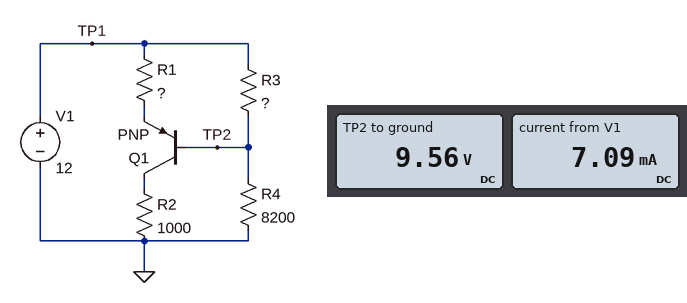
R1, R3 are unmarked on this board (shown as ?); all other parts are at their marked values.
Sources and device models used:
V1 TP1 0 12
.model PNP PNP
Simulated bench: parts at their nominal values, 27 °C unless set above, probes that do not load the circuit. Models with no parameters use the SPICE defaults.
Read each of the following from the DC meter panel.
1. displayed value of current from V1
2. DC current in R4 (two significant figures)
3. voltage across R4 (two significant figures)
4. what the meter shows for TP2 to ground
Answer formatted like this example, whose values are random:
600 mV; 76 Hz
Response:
7.09 mA; 1.2 mA; 9.6 V; 9.56 V
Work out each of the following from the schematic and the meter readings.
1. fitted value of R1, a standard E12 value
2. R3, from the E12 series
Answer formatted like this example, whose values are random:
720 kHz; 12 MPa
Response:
270 Ω; 2.2 kΩ
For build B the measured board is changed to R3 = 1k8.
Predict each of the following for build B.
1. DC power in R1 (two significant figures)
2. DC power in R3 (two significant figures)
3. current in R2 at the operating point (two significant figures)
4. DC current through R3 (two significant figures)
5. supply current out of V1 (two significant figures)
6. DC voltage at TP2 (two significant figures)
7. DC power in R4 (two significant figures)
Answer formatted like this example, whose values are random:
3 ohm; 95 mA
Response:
6.0 mW; 2.4 mW; 4.7 mA; 1.2 mA; 5.9 mA; 9.9 V; 12 mW
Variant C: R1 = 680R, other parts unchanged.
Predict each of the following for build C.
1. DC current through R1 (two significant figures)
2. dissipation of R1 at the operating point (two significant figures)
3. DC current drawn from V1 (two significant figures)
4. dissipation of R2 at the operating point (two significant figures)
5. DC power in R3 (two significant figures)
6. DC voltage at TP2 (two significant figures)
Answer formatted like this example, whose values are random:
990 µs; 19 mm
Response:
2.5 mA; 4.2 mW; 3.6 mA; 6.1 mW; 2.8 mW; 9.5 V
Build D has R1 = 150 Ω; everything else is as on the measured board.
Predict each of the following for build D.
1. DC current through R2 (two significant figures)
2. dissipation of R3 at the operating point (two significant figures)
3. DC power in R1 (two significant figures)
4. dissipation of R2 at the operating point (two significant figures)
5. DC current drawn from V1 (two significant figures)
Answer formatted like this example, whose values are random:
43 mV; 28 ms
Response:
10 mA; 2.5 mW; 16 mW; 100 mW; 11 mA
